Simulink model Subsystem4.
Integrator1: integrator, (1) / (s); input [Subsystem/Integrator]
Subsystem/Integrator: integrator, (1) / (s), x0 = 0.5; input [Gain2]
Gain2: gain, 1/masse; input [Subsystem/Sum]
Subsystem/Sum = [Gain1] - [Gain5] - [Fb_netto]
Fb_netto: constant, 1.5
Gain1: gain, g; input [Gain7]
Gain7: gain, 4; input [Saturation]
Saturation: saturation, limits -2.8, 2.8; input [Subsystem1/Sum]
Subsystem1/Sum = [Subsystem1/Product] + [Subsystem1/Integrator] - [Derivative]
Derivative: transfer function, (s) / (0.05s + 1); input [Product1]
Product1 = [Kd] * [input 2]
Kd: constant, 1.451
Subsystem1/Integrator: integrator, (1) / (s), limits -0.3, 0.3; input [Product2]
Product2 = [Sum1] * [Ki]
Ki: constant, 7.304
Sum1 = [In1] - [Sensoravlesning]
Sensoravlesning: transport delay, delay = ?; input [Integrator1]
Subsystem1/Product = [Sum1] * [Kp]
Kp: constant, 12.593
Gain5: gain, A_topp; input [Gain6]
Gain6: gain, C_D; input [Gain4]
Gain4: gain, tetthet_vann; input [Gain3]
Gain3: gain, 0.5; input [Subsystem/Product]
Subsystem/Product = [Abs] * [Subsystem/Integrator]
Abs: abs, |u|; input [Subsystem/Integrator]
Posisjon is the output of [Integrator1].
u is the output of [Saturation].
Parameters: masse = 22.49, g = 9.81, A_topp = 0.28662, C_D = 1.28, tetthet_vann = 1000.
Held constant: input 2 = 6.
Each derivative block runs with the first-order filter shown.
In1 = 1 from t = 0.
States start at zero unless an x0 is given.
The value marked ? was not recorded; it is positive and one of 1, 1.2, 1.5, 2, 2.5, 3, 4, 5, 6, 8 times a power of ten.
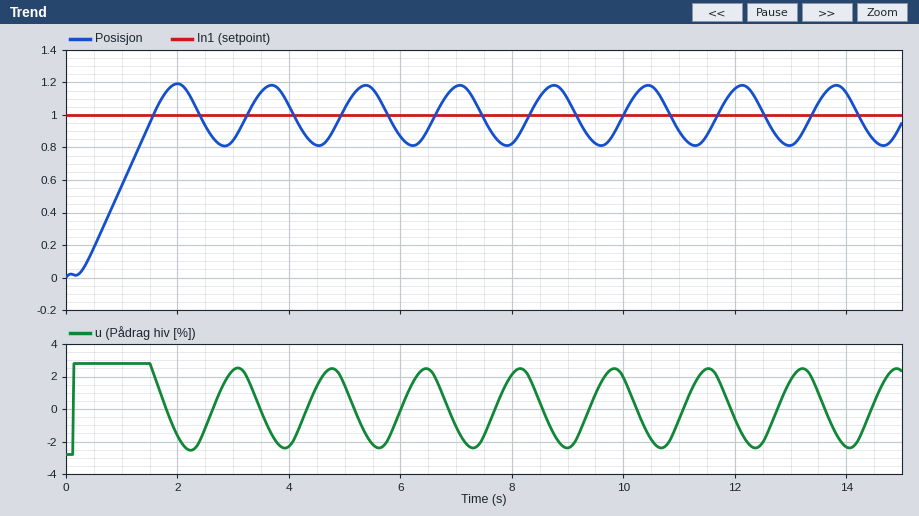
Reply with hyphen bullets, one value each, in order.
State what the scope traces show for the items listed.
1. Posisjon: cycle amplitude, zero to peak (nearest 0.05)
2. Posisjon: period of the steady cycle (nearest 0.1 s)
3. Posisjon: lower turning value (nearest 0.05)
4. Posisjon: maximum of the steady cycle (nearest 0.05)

- 0.20
- 1.7 s
- 0.80
- 1.20
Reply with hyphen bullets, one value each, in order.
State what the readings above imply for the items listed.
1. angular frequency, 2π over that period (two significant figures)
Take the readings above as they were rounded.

- 3.7 rad/s
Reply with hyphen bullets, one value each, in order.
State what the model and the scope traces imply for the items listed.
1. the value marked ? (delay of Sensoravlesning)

- 0.2
